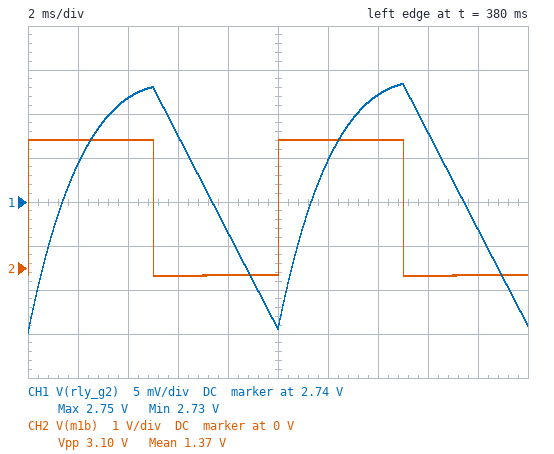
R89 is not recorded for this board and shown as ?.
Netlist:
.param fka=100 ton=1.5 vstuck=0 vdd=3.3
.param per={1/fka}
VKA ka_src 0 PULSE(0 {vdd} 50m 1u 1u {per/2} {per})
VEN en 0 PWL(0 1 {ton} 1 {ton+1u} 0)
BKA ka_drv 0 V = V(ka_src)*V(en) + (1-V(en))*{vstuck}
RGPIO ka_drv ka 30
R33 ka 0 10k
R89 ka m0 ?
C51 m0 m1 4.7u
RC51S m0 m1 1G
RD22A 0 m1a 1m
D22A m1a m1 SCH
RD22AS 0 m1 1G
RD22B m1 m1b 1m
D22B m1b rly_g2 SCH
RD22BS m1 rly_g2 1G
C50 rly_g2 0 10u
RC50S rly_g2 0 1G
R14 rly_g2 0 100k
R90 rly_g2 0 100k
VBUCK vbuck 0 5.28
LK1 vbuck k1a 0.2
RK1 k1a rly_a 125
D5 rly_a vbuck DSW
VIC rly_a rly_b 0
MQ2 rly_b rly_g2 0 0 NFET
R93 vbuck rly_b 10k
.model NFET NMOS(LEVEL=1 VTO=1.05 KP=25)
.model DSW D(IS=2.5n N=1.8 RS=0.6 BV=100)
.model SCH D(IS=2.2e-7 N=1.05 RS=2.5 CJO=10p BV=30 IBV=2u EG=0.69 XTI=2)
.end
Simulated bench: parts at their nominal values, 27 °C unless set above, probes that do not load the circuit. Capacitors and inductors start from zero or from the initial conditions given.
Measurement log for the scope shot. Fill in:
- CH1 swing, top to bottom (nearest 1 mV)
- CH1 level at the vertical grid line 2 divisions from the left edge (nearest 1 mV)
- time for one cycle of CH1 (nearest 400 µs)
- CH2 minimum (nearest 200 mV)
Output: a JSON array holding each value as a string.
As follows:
["28 mV", "2.752 V", "10.0 ms", "-200 mV"]
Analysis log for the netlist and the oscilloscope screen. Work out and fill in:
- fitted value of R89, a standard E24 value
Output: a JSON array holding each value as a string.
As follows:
["820 Ω"]
